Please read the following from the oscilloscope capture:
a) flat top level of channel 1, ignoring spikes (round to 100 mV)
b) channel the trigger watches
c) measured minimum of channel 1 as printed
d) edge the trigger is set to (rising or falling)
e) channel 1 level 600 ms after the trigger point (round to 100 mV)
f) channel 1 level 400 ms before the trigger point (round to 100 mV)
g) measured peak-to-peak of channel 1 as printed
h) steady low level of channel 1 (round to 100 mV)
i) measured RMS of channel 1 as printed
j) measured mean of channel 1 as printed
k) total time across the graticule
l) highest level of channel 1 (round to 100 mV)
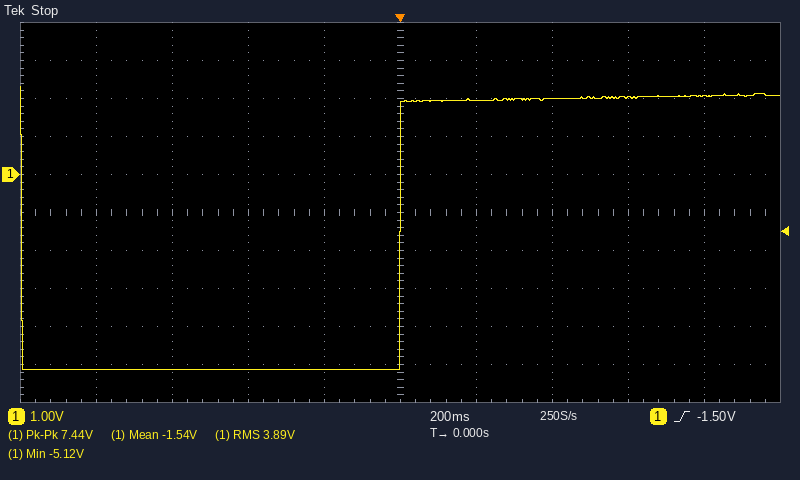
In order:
2.0 V
channel 1
-5.12 V
rising
2.0 V
-5.1 V
7.44 V
-5.1 V
3.89 V
-1.54 V
2 s
2.3 V
